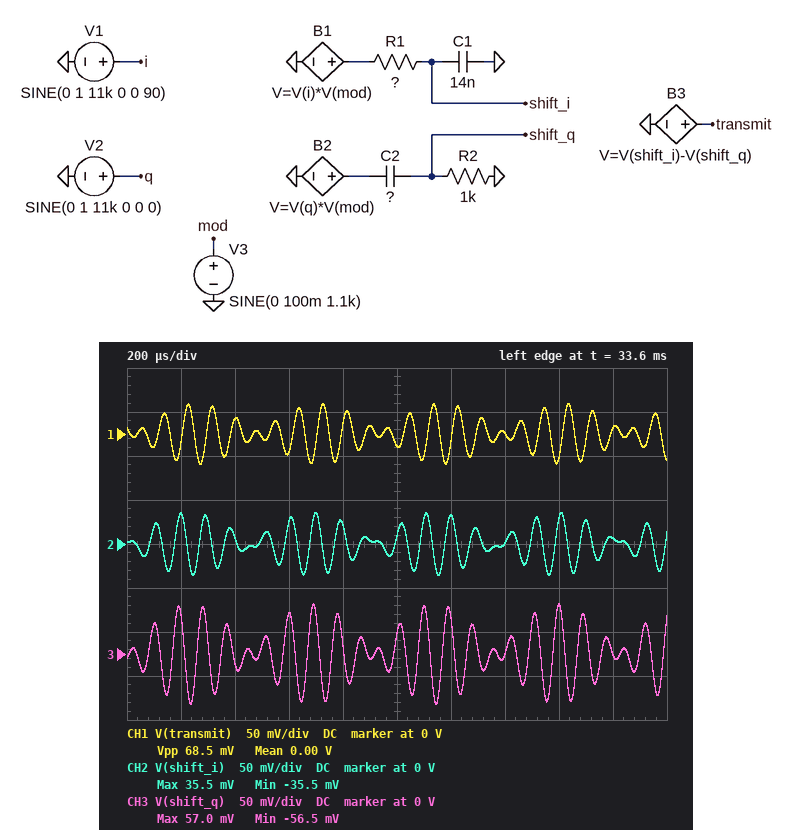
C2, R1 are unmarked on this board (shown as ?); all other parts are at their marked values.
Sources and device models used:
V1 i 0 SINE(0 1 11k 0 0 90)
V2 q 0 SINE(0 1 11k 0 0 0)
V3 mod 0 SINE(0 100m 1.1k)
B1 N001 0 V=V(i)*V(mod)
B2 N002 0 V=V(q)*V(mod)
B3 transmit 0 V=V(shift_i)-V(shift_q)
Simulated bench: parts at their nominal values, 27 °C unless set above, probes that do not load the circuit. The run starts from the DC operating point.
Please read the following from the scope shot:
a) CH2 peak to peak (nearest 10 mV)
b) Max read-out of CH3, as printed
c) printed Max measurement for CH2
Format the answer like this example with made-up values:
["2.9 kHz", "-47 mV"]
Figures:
["70 mV", "57.0 mV", "35.5 mV"]
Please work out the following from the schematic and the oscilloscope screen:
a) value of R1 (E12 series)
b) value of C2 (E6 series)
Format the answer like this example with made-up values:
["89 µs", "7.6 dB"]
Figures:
["2.7 kΩ", "10 nF"]
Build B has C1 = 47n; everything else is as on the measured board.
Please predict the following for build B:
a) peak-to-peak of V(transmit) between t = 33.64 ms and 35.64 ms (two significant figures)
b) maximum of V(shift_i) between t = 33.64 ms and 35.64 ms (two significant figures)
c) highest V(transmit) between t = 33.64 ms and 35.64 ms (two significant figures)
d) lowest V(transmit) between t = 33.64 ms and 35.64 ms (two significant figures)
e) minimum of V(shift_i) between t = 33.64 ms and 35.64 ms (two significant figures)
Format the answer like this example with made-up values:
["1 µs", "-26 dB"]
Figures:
["100 mV", "11 mV", "50 mV", "-50 mV", "-11 mV"]
